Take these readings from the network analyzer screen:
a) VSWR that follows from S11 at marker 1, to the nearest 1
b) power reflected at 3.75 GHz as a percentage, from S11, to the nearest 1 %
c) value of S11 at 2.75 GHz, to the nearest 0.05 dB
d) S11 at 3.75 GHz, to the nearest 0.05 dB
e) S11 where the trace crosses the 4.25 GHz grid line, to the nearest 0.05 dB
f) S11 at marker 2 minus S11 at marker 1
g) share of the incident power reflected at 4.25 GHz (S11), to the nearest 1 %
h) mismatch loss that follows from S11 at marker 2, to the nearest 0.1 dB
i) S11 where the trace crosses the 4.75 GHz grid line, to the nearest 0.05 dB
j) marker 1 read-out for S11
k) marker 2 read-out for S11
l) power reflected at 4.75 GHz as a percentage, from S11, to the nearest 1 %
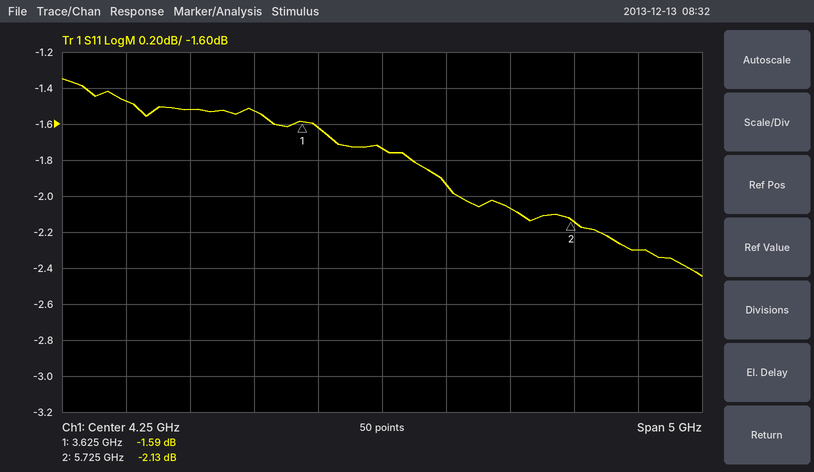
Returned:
11
69 %
-1.50 dB
-1.60 dB
-1.75 dB
-0.54 dB
67 %
4.1 dB
-1.95 dB
-1.59 dB
-2.13 dB
64 %
